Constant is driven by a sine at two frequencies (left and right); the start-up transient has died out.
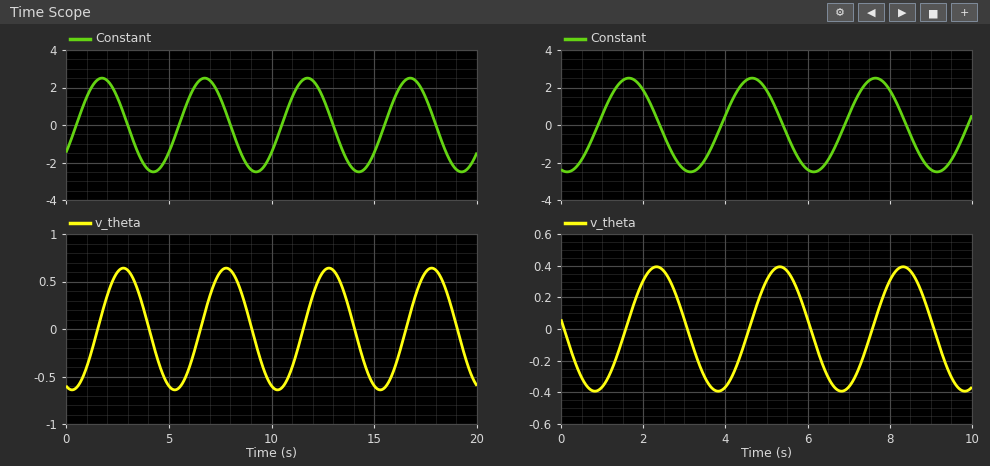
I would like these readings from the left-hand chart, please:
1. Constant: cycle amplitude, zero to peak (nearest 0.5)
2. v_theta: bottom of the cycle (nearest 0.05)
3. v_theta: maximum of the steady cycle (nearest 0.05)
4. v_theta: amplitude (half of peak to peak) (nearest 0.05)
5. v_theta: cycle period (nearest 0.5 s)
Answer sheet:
2.5
-0.65
0.65
0.65
5.0 s
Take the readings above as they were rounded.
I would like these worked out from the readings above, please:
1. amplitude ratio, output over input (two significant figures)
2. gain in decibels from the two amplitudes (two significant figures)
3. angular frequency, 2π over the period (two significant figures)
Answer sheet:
0.26
-12 dB
1.3 rad/s
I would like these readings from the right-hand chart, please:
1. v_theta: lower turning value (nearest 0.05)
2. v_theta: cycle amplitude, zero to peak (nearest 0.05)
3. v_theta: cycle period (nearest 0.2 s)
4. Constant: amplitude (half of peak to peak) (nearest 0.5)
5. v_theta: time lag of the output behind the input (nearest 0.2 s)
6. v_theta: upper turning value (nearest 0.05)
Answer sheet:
-0.40
0.40
3.0 s
2.5
0.6 s
0.40
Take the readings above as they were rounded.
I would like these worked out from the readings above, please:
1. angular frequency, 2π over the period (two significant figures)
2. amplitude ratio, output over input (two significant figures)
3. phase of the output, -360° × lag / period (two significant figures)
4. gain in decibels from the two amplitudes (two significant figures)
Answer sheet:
2.1 rad/s
0.16
-72°
-16 dB
